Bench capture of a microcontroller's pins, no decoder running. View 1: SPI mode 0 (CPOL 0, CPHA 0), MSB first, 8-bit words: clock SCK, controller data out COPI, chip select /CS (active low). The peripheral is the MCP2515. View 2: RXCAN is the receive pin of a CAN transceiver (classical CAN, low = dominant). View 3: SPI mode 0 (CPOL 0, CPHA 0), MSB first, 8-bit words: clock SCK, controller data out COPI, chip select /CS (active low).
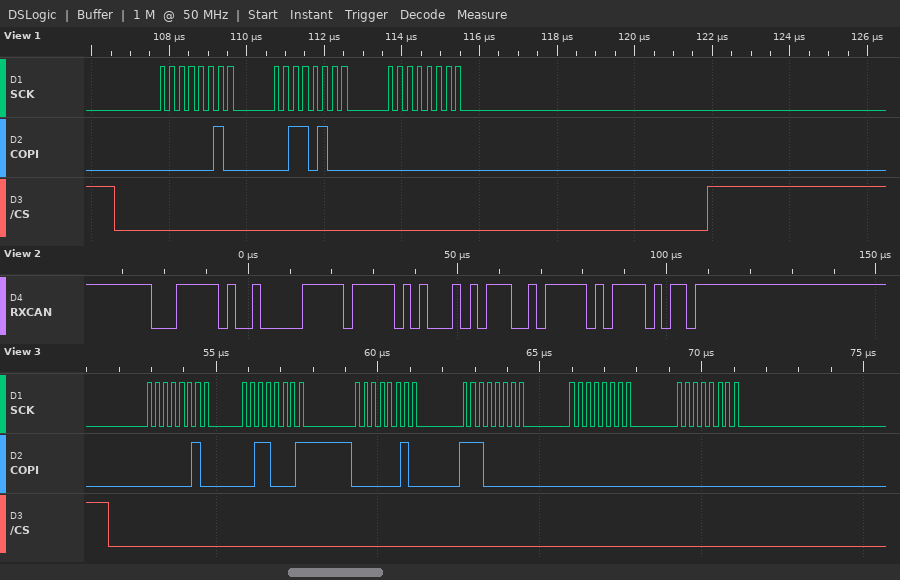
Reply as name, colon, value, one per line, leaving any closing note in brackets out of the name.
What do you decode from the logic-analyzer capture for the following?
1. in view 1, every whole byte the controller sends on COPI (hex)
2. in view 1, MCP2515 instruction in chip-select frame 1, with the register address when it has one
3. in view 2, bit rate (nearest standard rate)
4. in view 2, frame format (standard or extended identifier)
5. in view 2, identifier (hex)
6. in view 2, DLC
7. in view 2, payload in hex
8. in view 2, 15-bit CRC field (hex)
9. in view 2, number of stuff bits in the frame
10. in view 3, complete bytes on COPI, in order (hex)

in view 1, every whole byte the controller sends on COPI: 02 34 00
in view 1, MCP2515 instruction in chip-select frame 1, with the register address when it has one: WRITE 0x34
in view 2, bit rate: 500 kbit/s
in view 2, frame format: standard
in view 2, identifier: 0x1F9
in view 2, DLC: 3
in view 2, payload in hex: FF 45 72
in view 2, 15-bit CRC field: 0x7EF5
in view 2, number of stuff bits in the frame: 5
in view 3, complete bytes on COPI, in order: 0x02 0x31 0x02 0xE0 0x00 0x00
